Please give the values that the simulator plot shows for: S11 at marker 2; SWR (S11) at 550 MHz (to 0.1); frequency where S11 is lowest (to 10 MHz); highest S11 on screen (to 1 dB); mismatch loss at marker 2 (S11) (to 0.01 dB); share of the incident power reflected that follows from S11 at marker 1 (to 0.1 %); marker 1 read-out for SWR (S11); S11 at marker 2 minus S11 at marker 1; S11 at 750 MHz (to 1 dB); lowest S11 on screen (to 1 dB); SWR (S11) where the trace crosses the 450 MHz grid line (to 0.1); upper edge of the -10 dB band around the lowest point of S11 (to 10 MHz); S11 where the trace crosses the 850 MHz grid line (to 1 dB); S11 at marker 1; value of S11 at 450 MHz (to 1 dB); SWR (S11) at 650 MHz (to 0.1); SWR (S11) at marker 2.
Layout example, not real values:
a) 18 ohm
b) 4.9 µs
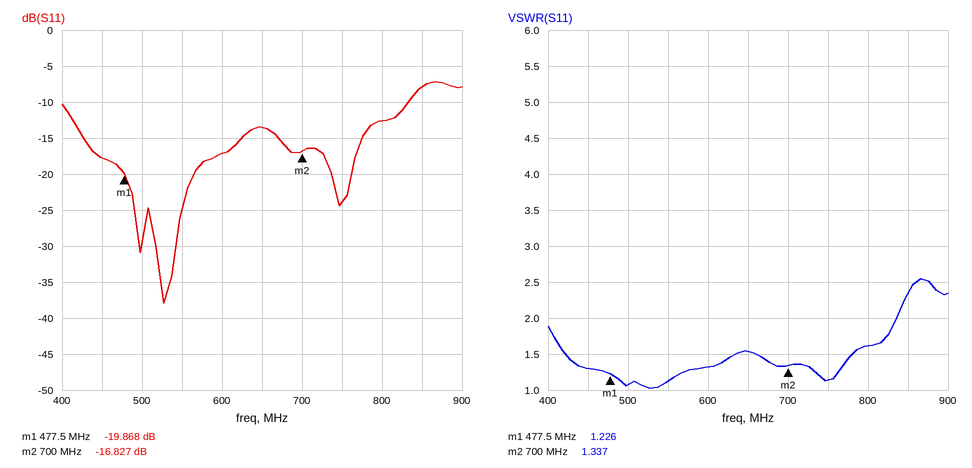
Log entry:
a) -16.827 dB
b) 1.1
c) 530 MHz
d) -7 dB
e) 0.09 dB
f) 1.0 %
g) 1.226
h) 3.041 dB
i) -24 dB
j) -38 dB
k) 1.3
l) 830 MHz
m) -8 dB
n) -19.868 dB
o) -18 dB
p) 1.5
q) 1.337
